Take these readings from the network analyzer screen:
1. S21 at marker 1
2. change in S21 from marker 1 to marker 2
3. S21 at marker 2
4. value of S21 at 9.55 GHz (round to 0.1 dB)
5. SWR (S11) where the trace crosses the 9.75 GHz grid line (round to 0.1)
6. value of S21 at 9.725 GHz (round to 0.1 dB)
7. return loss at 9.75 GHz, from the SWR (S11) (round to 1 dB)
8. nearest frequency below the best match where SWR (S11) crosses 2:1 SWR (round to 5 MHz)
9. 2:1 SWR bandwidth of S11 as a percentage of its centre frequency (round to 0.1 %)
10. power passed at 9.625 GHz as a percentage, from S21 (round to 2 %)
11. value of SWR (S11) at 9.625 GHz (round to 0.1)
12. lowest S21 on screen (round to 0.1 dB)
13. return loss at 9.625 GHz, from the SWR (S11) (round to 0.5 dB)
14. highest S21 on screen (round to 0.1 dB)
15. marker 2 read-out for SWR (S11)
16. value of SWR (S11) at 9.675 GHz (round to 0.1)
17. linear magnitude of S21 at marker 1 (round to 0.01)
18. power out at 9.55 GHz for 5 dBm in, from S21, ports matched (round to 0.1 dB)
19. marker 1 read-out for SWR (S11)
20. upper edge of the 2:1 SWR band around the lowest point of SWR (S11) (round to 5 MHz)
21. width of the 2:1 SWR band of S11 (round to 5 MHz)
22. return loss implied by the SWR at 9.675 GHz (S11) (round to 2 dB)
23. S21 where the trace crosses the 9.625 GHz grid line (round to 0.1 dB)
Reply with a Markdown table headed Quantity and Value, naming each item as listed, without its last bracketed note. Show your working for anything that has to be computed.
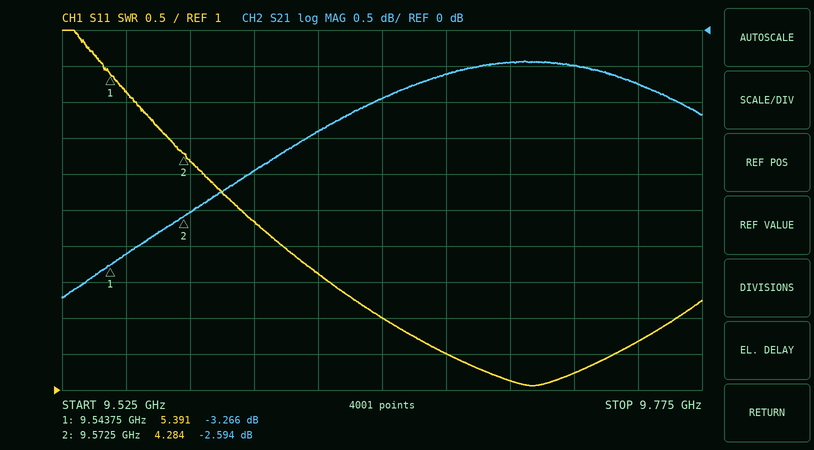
| Quantity | Value |
|---|---|
| S21 at marker 1 | -3.266 dB |
| change in S21 from marker 1 to marker 2 | -2.594 − (-3.266) = 0.672 dB |
| S21 at marker 2 | -2.594 dB |
| value of S21 at 9.55 GHz | -3.1 dB |
| SWR (S11) where the trace crosses the 9.75 GHz grid line | 1.7 |
| value of S21 at 9.725 GHz | -0.5 dB |
| return loss at 9.75 GHz, from the SWR (S11) | −20 log10((1.7 − 1)/(1.7 + 1)) ≈ 12 dB |
| nearest frequency below the best match where SWR (S11) crosses 2:1 SWR | 9.650 GHz |
| 2:1 SWR bandwidth of S11 as a percentage of its centre frequency | 115 MHz / 9.7075 GHz ≈ 1.2 % |
| power passed at 9.625 GHz as a percentage, from S21 | 10^(-1.4/10) ≈ 72 % |
| value of SWR (S11) at 9.625 GHz | 2.6 |
| lowest S21 on screen | -3.7 dB |
| return loss at 9.625 GHz, from the SWR (S11) | −20 log10((2.6 − 1)/(2.6 + 1)) ≈ 7.0 dB |
| highest S21 on screen | -0.4 dB |
| marker 2 read-out for SWR | 4.284 |
| value of SWR (S11) at 9.675 GHz | 1.5 |
| linear magnitude of S21 at marker 1 | 10^(-3.266/20) ≈ 0.69 |
| power out at 9.55 GHz for 5 dBm in, from S21, ports matched | 5 dBm + (-3.1 dB) = 1.9 dBm |
| marker 1 read-out for SWR | 5.391 |
| upper edge of the 2:1 SWR band around the lowest point of SWR (S11) | 9.765 GHz |
| width of the 2:1 SWR band of S11 | 9.765 GHz − 9.650 GHz = 115 MHz |
| return loss implied by the SWR at 9.675 GHz (S11) | −20 log10((1.5 − 1)/(1.5 + 1)) ≈ 14 dB |
| S21 where the trace crosses the 9.625 GHz grid line | -1.4 dB |
